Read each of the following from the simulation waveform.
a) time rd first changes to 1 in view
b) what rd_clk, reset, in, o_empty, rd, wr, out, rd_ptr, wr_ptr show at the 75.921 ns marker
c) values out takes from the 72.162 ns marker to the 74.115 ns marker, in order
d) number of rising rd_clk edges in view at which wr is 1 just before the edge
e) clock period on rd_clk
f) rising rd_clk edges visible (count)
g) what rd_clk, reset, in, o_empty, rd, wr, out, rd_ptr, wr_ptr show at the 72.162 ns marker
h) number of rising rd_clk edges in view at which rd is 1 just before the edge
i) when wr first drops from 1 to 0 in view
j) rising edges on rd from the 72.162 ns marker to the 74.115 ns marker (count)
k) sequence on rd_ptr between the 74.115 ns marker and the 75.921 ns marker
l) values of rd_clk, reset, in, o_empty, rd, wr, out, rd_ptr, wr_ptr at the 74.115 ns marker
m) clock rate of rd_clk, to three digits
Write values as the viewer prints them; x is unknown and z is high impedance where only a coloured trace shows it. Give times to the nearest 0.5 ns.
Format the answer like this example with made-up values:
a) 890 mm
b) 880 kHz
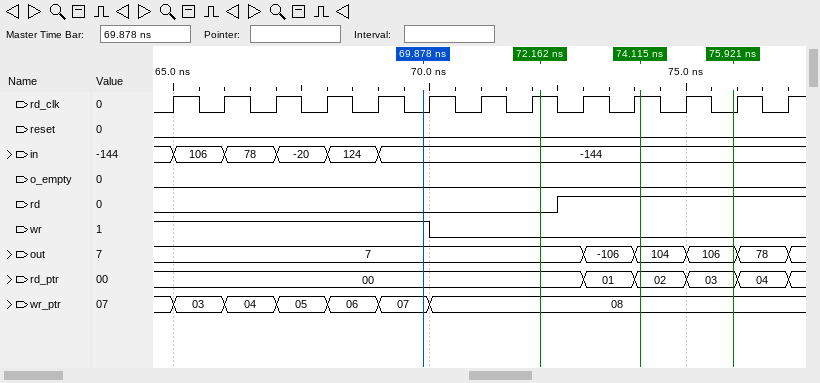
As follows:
a) 72.5 ns
b) rd_clk=0, reset=0, in=-144, o_empty=0, rd=1, wr=0, out=106, rd_ptr=03, wr_ptr=08
c) 7, -106, 104
d) 6
e) 1 ns
f) 13
g) rd_clk=1, reset=0, in=-144, o_empty=0, rd=0, wr=0, out=7, rd_ptr=00, wr_ptr=08
h) 5
i) 70 ns
j) 1
k) 02, 03
l) rd_clk=1, reset=0, in=-144, o_empty=0, rd=1, wr=0, out=104, rd_ptr=02, wr_ptr=08
m) 1.00 GHz
